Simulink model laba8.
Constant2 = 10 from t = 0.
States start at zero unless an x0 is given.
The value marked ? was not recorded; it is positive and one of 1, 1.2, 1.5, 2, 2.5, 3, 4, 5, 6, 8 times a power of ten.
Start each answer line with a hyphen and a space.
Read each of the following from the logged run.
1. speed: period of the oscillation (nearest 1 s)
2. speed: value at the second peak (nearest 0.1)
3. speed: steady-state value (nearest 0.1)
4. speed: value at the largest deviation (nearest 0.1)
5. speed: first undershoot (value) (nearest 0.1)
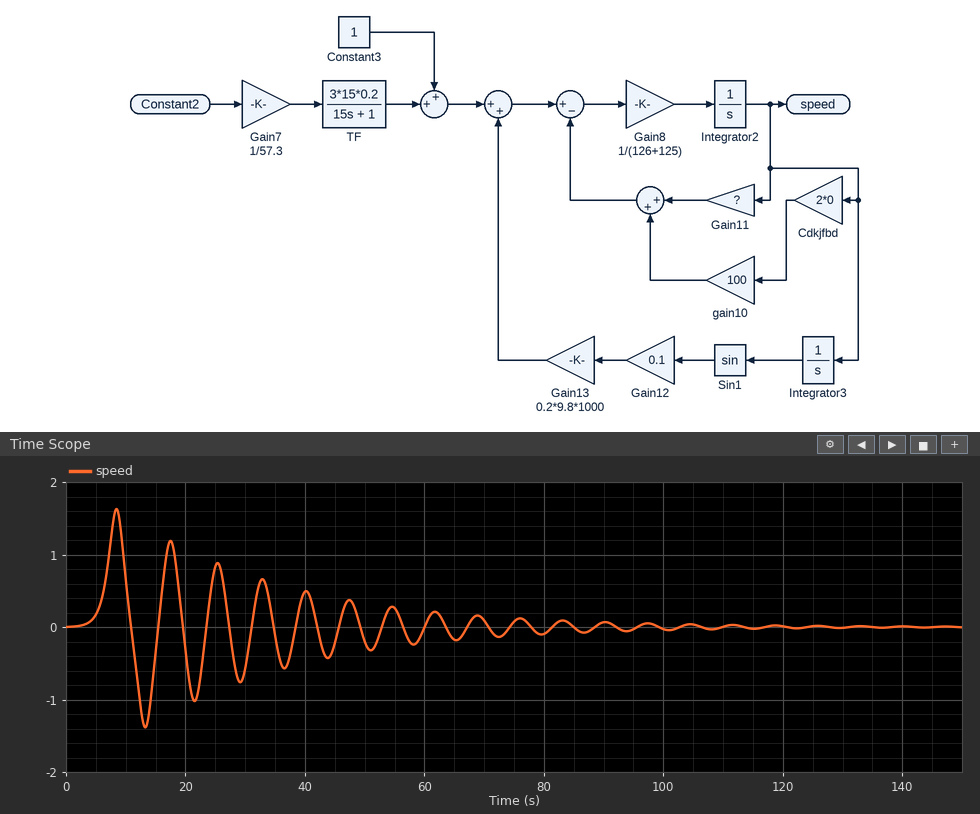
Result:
- 9 s
- 1.2
- 0.0
- 1.6
- -1.4
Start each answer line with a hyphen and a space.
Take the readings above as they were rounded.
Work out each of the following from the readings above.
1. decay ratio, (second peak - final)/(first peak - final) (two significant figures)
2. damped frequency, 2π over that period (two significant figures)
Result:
- 0.75
- 0.70 rad/s
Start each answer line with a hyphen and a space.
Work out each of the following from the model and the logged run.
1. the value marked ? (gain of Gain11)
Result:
- 20
